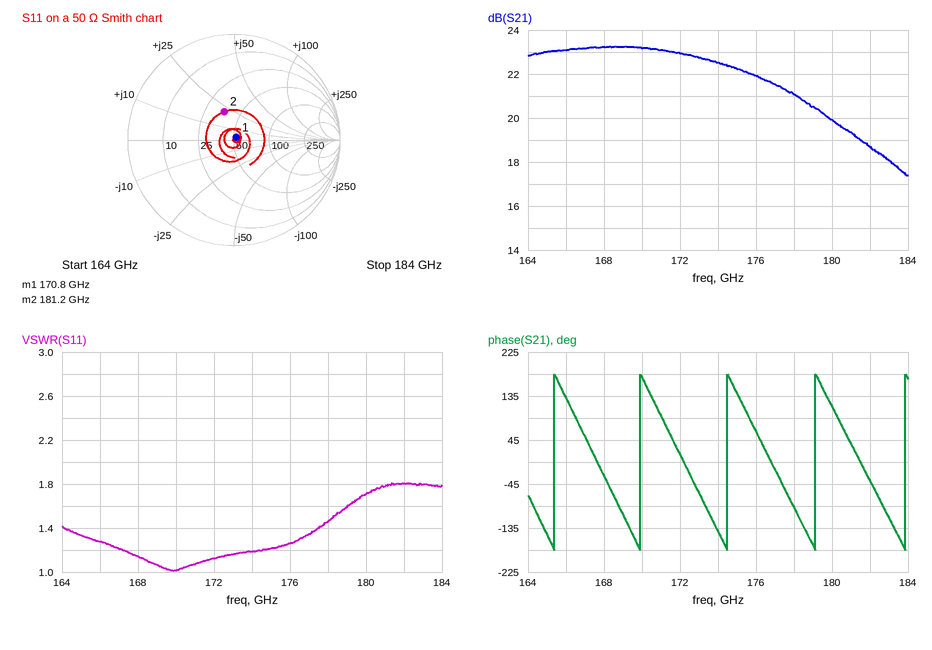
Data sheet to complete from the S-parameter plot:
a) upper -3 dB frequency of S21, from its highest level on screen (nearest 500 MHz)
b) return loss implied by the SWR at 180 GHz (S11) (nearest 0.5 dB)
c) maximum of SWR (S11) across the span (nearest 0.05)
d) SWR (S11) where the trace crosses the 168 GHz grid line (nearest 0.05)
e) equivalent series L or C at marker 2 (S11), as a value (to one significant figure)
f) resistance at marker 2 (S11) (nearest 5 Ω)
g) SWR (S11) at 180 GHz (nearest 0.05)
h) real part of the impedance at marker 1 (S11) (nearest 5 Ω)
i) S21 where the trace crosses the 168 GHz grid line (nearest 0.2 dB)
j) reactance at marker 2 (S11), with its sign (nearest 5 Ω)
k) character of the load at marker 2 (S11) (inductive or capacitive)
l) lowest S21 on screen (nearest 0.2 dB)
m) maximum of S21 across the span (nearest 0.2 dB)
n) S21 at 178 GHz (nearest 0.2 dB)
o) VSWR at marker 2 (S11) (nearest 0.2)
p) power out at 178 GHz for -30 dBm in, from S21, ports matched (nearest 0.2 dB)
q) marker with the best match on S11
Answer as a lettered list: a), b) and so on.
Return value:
a) 179.5 GHz
b) 11.5 dB
c) 1.80
d) 1.15
e) 20 pH
f) 35 Ω
g) 1.70
h) 50 Ω
i) 23.2 dB
j) +20 Ω
k) inductive
l) 17.4 dB
m) 23.2 dB
n) 21.0 dB
o) 1.8
p) -9.0 dBm
q) marker 1
